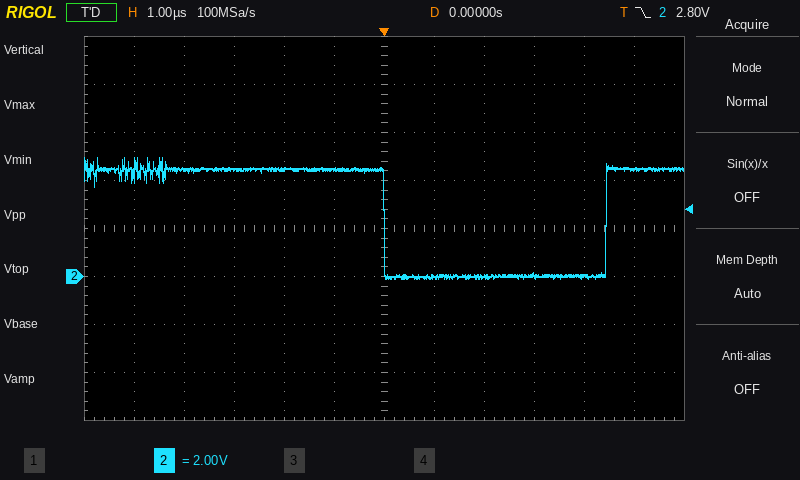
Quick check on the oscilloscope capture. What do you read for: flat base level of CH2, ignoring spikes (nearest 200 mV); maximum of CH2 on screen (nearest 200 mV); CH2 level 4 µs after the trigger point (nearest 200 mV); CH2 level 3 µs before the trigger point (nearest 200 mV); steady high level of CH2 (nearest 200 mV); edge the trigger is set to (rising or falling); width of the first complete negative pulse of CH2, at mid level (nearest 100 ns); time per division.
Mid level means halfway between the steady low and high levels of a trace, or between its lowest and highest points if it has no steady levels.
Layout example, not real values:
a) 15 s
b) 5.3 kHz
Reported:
a) 0.0 V
b) 5.0 V
c) 0.0 V
d) 4.4 V
e) 4.4 V
f) falling
g) 4.4 µs
h) 1 µs
